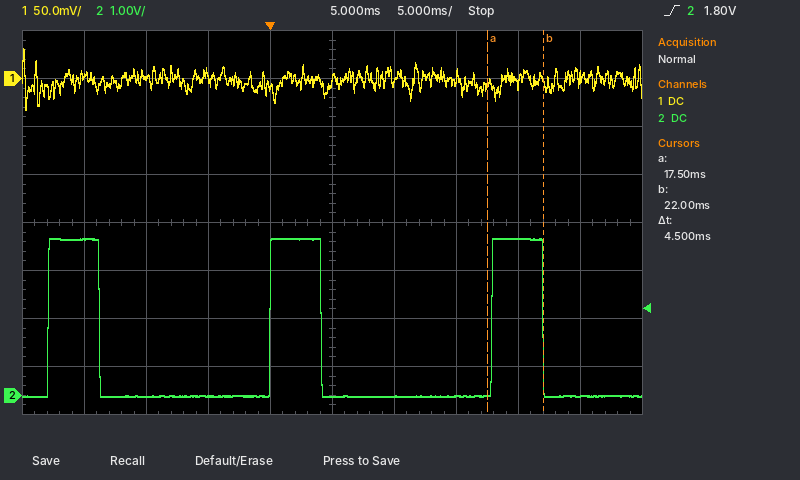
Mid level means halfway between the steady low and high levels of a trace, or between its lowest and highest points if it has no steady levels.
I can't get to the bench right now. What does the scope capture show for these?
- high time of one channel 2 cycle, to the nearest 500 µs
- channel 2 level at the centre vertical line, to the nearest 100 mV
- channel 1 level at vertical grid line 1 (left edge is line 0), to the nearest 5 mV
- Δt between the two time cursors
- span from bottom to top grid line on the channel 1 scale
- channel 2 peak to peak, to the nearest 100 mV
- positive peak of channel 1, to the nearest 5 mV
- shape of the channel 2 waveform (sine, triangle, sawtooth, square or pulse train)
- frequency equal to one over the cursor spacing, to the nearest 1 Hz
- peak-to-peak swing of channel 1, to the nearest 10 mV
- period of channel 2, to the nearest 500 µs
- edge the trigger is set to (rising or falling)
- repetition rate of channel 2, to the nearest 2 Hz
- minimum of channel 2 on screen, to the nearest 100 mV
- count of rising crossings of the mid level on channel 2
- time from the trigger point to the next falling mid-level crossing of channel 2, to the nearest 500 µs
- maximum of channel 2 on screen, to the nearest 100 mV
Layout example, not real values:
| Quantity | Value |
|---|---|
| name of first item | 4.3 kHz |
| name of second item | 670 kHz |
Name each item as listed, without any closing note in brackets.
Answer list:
| Quantity | Value |
|---|---|
| high time of one channel 2 cycle, to the nearest 500 µs | 4.0 ms |
| channel 2 level at the centre vertical line, to the nearest 100 mV | 0.0 V |
| channel 1 level at vertical grid line 1 (left edge is line 0), to the nearest 5 mV | 5 mV |
| Δt between the two time cursors | 4.5 ms |
| span from bottom to top grid line on the channel 1 scale | 400 mV |
| channel 2 peak to peak, to the nearest 100 mV | 3.3 V |
| positive peak of channel 1, to the nearest 5 mV | 30 mV |
| shape of the channel 2 waveform | pulse train |
| frequency equal to one over the cursor spacing, to the nearest 1 Hz | 222 Hz |
| peak-to-peak swing of channel 1, to the nearest 10 mV | 60 mV |
| period of channel 2, to the nearest 500 µs | 18.0 ms |
| edge the trigger is set to | rising |
| repetition rate of channel 2, to the nearest 2 Hz | 56 Hz |
| minimum of channel 2 on screen, to the nearest 100 mV | 0.0 V |
| count of rising crossings of the mid level on channel 2 | 3 |
| time from the trigger point to the next falling mid-level crossing of channel 2, to the nearest 500 µs | 4.0 ms |
| maximum of channel 2 on screen, to the nearest 100 mV | 3.3 V |
